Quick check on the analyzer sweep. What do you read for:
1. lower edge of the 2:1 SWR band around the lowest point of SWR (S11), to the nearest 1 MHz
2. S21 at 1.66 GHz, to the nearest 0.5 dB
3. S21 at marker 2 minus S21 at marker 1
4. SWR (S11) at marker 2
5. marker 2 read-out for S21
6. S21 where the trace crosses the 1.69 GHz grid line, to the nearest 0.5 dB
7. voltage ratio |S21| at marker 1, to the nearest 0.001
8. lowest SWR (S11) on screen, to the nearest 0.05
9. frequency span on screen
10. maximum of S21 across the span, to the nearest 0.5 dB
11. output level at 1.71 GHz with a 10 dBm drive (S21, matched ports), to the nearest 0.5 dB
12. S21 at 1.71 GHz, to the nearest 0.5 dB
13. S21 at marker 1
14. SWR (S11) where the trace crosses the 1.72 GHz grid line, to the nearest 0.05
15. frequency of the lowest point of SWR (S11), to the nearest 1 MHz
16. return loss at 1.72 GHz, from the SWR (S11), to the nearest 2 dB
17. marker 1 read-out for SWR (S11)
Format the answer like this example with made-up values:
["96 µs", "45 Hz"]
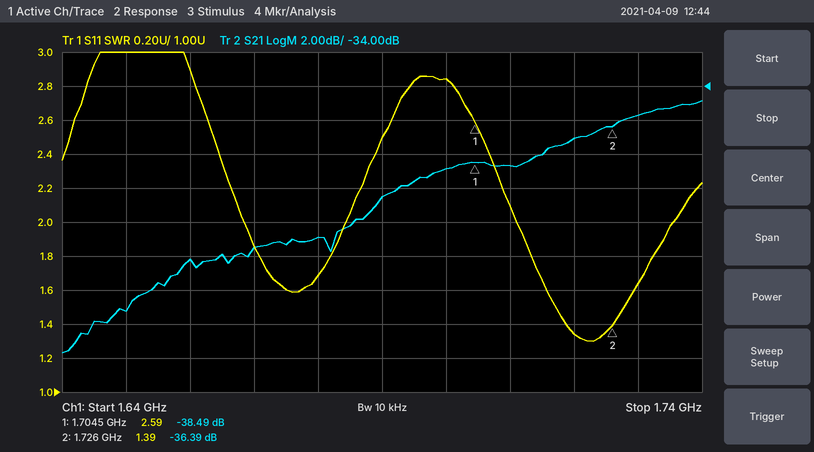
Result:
["1.711 GHz", "-44.0 dB", "2.10 dB", "1.39", "-36.39 dB", "-40.5 dB", "0.012", "1.30", "100 MHz", "-35.0 dB", "-28.5 dBm", "-38.5 dB", "-38.49 dB", "1.35", "1.723 GHz", "16 dB", "2.59"]
